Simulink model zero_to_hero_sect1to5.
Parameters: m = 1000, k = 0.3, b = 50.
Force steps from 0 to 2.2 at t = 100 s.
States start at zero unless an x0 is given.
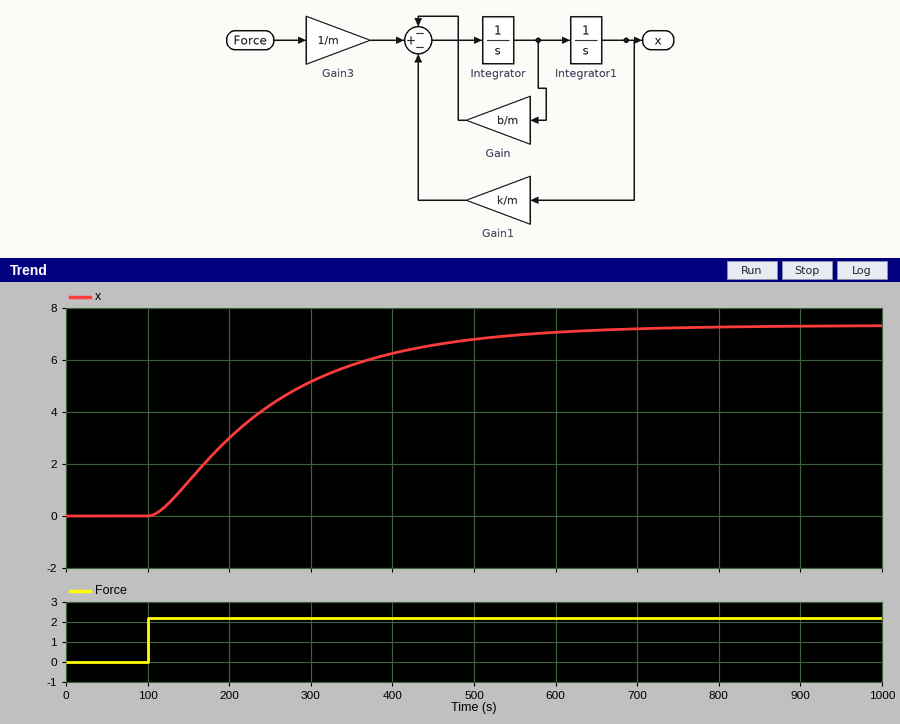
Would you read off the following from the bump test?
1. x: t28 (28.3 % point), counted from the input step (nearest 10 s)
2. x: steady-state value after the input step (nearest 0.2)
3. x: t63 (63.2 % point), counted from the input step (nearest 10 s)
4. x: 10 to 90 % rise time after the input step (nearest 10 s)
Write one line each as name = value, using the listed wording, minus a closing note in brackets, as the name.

x: t28 (28.3 % point), counted from the input step = 70 s
x: steady-state value after the input step = 7.4
x: t63 (63.2 % point), counted from the input step = 170 s
x: 10 to 90 % rise time after the input step = 320 s
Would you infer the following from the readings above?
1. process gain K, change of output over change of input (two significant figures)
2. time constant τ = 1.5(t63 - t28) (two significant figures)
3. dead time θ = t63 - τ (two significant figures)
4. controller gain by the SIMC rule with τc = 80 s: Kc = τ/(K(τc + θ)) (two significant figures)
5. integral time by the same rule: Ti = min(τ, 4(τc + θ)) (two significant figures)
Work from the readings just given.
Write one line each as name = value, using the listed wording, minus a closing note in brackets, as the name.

process gain K, change of output over change of input = 3.4
time constant τ = 1.5(t63 - t28) = 150 s
dead time θ = t63 - τ = 20 s
controller gain by the SIMC rule with τc = 80 s: Kc = τ/(K(τc + θ)) = 0.44
integral time by the same rule: Ti = min(τ, 4(τc + θ)) = 150 s
